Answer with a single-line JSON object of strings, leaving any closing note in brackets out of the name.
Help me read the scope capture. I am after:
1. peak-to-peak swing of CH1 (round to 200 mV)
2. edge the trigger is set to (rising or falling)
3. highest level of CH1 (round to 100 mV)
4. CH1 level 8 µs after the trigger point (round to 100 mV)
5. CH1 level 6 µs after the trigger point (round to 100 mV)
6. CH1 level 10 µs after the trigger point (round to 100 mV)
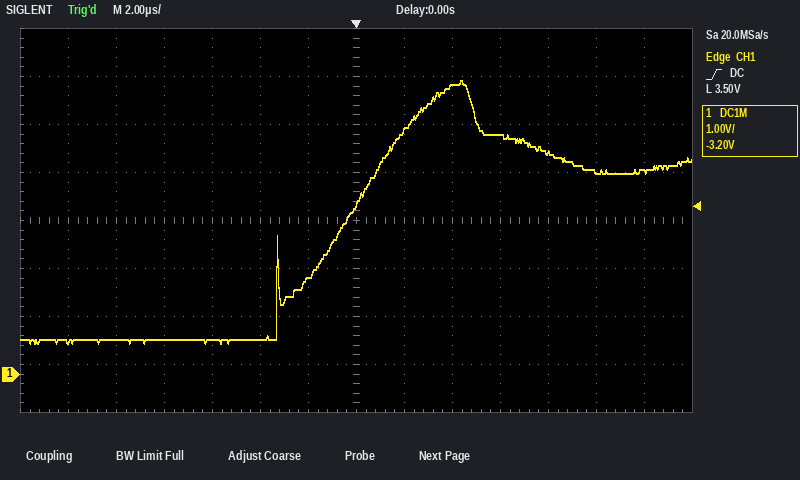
{"peak-to-peak swing of CH1": "5.4 V", "edge the trigger is set to": "rising", "highest level of CH1": "6.1 V", "CH1 level 8 µs after the trigger point": "4.6 V", "CH1 level 6 µs after the trigger point": "5.0 V", "CH1 level 10 µs after the trigger point": "4.2 V"}
